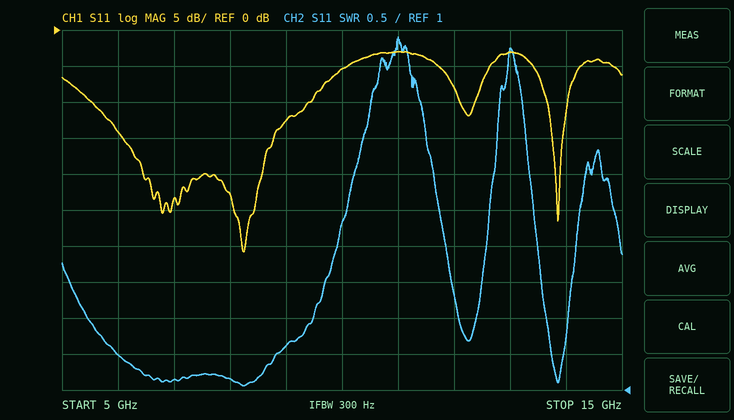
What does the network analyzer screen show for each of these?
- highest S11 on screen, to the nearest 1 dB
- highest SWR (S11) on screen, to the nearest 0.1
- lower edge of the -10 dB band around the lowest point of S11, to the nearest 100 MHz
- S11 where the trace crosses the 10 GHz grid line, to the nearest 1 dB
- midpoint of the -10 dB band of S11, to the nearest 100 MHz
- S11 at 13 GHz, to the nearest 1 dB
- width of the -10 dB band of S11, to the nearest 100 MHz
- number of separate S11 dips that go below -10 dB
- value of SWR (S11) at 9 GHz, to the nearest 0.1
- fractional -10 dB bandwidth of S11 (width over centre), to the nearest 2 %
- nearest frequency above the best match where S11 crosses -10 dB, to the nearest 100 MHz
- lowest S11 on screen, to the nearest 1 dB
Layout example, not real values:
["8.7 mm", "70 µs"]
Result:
["-3 dB", "5.9", "5.5 GHz", "-5 dB", "7.5 GHz", "-3 dB", "3.9 GHz", "4", "1.6", "52 %", "9.4 GHz", "-31 dB"]
